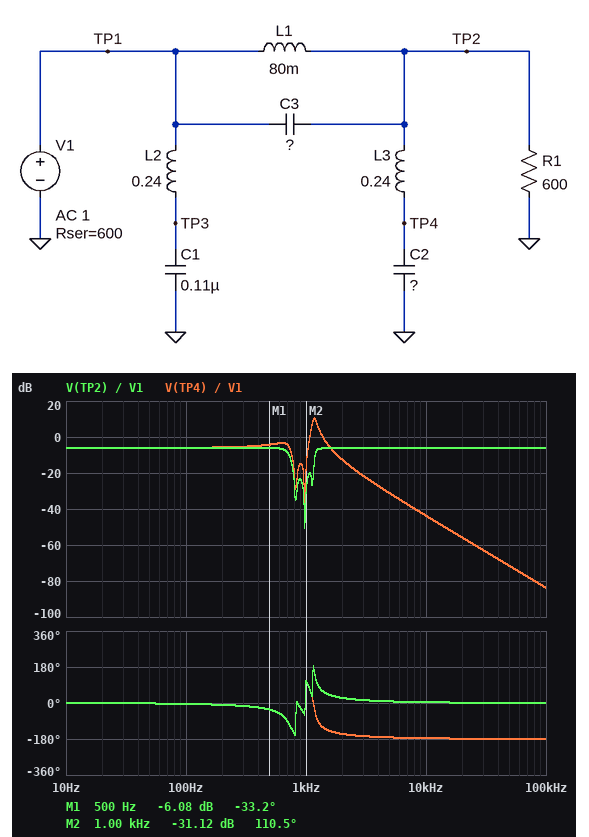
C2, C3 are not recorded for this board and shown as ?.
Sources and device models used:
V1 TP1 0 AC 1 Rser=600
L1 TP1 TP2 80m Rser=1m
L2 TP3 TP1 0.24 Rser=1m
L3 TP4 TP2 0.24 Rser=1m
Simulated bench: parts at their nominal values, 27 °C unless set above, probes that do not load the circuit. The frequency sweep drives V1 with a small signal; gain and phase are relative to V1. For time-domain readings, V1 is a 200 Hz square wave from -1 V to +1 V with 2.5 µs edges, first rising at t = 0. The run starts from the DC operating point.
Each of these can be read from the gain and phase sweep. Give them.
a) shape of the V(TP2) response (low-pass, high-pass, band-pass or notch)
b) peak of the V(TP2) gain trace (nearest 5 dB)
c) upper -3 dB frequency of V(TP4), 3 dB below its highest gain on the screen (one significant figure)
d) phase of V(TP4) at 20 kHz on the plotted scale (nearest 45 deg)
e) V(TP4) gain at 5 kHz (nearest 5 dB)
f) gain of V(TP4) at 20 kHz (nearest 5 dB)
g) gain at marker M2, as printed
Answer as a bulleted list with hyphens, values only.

- notch
- -5 dB
- 1 kHz
- -180 deg
- -30 dB
- -55 dB
- -31.12 dB
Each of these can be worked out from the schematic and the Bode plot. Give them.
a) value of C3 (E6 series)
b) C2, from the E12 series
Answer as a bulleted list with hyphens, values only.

- 470 nF
- 82 nF
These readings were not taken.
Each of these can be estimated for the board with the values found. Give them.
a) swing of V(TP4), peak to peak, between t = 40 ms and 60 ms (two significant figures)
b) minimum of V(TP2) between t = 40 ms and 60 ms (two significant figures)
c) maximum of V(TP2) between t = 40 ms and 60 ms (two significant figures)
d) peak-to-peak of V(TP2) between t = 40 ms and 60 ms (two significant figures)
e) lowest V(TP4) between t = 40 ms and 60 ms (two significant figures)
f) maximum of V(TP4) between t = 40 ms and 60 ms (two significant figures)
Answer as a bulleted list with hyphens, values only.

- 1.5 V
- -720 mV
- 720 mV
- 1.4 V
- -770 mV
- 770 mV
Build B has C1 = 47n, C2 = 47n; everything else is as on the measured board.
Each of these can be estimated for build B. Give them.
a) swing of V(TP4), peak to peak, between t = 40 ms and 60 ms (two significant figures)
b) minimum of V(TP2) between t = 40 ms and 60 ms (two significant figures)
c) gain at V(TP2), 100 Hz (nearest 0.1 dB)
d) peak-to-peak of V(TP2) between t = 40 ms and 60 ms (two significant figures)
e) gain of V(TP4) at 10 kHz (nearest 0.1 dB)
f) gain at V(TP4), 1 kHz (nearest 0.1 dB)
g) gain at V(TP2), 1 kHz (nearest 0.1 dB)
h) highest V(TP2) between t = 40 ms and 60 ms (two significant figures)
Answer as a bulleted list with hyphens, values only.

- 1.8 V
- -650 mV
- -6.0 dB
- 1.3 V
- -38.8 dB
- -5.1 dB
- -10.2 dB
- 650 mV
